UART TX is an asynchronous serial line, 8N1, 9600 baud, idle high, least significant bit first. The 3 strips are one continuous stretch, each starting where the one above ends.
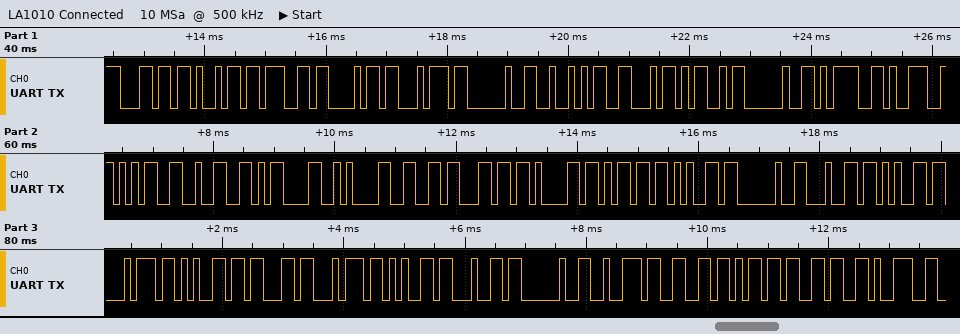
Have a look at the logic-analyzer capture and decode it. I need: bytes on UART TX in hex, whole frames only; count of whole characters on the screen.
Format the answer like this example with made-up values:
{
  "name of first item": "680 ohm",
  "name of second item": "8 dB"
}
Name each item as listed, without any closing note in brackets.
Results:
{
  "bytes on UART TX in hex, whole frames only": "6C 69 67 68 74 20 52 46 4D 20 3D 39 35 32 0D 0A 66 6C 61 6D 65 20 64 65 74 65 63 74 65 64 20 72 66 6D 36 39",
  "count of whole characters on the screen": "36"
}
